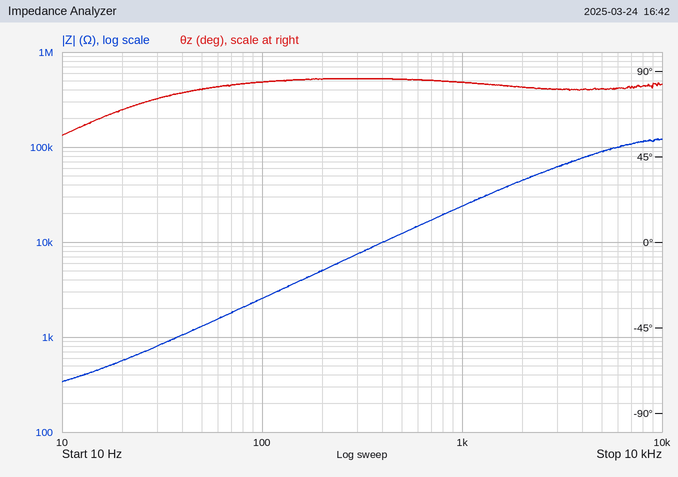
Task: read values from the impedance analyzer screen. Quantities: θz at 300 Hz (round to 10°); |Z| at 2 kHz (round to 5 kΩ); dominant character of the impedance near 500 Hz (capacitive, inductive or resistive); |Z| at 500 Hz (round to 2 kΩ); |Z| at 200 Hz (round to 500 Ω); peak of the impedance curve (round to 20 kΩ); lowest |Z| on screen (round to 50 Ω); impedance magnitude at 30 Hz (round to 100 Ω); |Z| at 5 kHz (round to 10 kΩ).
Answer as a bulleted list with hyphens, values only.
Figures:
- 90°
- 45 kΩ
- inductive
- 12 kΩ
- 5.0 kΩ
- 120 kΩ
- 350 Ω
- 800 Ω
- 90 kΩ
